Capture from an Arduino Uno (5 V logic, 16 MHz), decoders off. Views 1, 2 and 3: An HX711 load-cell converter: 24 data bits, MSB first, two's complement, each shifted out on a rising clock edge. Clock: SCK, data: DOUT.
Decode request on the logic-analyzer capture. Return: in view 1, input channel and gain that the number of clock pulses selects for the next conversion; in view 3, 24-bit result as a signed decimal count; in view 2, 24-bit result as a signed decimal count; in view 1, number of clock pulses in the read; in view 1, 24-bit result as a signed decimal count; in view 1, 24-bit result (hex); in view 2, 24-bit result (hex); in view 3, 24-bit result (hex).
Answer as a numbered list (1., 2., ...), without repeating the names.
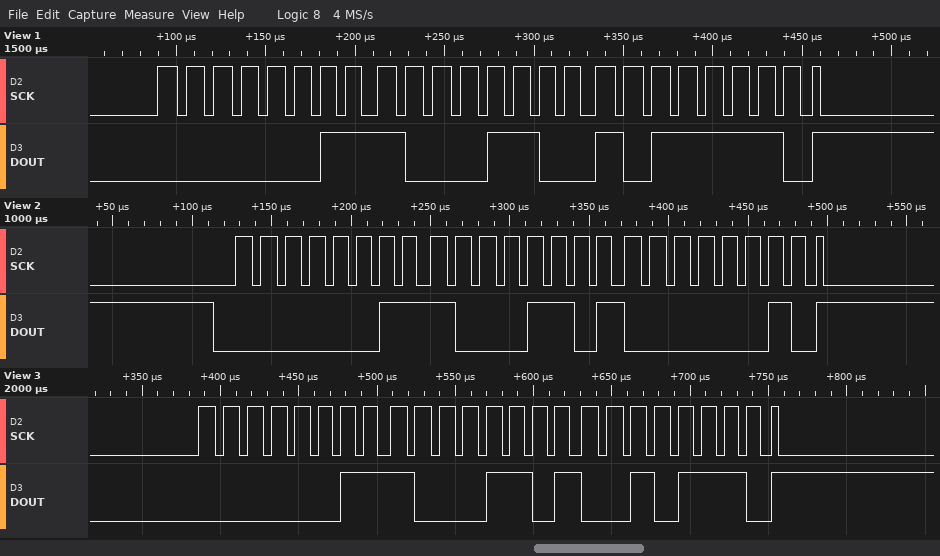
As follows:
1. channel A, gain 128
2. 232750
3. 232706
4. 25
5. 232638
6. 0x038CBE
7. 0x038D02
8. 0x038D2E
